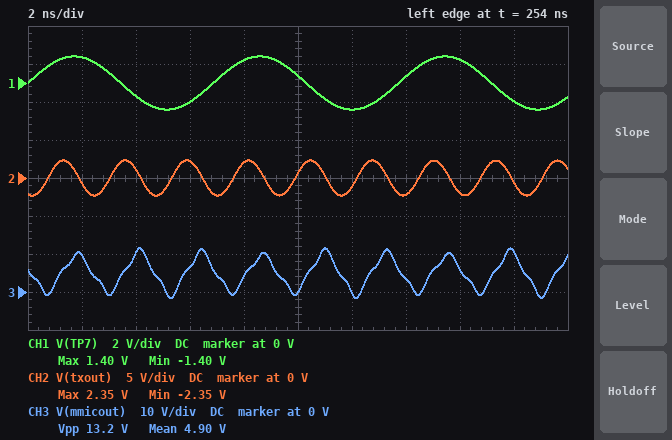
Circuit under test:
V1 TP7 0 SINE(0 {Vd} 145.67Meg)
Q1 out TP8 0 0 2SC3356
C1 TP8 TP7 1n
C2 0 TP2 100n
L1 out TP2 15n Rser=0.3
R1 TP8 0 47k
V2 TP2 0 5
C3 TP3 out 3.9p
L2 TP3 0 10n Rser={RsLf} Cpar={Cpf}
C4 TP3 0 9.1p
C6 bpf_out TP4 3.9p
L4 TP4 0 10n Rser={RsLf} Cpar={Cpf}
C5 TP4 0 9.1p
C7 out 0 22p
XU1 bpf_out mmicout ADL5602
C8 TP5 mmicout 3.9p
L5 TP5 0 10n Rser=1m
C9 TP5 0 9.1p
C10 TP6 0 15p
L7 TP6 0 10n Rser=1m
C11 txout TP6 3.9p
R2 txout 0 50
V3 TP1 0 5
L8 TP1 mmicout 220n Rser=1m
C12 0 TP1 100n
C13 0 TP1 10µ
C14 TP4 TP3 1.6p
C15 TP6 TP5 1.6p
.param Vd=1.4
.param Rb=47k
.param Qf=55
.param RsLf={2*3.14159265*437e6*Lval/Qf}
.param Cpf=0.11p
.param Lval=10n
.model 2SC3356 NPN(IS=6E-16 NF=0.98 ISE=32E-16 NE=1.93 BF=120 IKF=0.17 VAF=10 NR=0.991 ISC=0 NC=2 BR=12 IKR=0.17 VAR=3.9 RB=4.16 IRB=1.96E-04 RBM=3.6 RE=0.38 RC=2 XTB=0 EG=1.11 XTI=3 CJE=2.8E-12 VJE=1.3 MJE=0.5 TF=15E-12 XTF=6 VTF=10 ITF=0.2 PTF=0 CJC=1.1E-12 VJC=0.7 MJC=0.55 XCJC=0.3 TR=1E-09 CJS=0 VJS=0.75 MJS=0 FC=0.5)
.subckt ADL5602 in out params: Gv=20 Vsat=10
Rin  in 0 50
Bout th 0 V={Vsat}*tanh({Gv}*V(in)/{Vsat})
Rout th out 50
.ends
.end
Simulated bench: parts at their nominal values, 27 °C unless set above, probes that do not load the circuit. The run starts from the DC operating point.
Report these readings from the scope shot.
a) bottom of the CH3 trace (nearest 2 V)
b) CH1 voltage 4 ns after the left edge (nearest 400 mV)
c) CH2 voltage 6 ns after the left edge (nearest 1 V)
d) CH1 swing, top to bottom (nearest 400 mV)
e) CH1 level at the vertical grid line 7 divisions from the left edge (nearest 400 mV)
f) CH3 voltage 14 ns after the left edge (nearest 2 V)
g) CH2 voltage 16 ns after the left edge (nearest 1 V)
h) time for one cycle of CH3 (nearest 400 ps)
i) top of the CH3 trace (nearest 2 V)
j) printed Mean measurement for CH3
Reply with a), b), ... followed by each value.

a) -2 V
b) -800 mV
c) 2 V
d) 2.8 V
e) 400 mV
f) 4 V
g) -2 V
h) 2.4 ns
i) 12 V
j) 4.90 V
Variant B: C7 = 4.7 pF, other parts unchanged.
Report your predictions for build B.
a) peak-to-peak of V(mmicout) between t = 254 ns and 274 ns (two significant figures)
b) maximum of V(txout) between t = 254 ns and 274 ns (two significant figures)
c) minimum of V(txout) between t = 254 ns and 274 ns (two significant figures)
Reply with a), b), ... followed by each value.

a) 18 V
b) 2.5 V
c) -2.5 V
